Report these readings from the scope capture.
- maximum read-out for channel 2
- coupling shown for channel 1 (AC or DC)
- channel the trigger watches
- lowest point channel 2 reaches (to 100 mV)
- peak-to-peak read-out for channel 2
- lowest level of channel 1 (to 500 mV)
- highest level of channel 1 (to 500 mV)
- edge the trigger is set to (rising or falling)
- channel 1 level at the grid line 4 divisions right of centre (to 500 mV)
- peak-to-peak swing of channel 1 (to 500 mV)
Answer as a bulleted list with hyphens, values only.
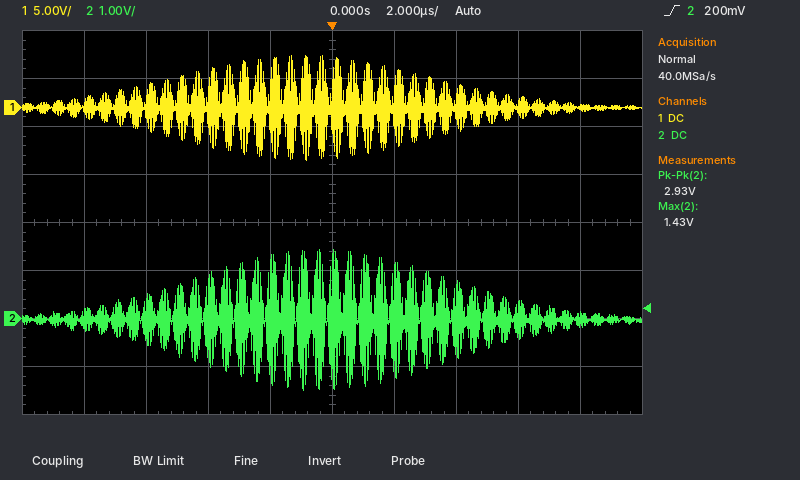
- 1.43 V
- DC
- channel 2
- -1.5 V
- 2.93 V
- -5.5 V
- 5.5 V
- rising
- 0.0 V
- 11.0 V
